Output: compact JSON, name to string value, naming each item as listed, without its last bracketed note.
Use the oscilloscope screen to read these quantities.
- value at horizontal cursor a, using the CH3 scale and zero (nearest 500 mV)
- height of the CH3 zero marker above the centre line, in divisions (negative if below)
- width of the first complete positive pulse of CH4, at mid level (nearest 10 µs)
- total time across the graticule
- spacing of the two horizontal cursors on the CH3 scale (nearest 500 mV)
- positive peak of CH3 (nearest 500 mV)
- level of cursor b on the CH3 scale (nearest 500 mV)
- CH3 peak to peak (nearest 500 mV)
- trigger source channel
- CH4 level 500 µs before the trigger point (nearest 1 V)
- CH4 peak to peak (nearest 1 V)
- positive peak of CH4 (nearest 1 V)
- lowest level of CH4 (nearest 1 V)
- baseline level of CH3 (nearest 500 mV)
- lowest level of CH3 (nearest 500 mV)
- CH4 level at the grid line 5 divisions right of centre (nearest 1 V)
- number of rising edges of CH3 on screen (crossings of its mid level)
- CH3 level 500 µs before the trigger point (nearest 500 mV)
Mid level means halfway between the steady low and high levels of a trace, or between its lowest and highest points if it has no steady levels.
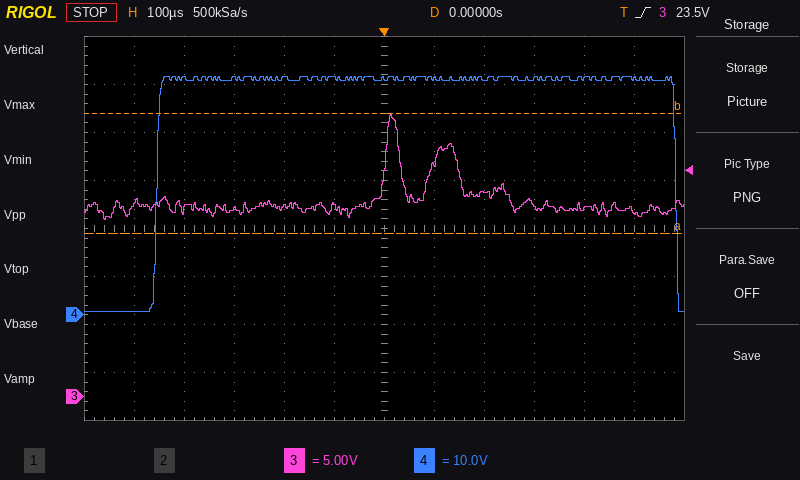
{"value at horizontal cursor a, using the CH3 scale and zero": "17.0 V", "height of the CH3 zero marker above the centre line, in divisions": "-3.5 div", "width of the first complete positive pulse of CH4, at mid level": "1.04 ms", "total time across the graticule": "1.2 ms", "spacing of the two horizontal cursors on the CH3 scale": "12.5 V", "positive peak of CH3": "29.5 V", "level of cursor b on the CH3 scale": "29.5 V", "CH3 peak to peak": "11.0 V", "trigger source channel": "CH3", "CH4 level 500 µs before the trigger point": "1 V", "CH4 peak to peak": "49 V", "positive peak of CH4": "50 V", "lowest level of CH4": "1 V", "baseline level of CH3": "19.5 V", "lowest level of CH3": "18.5 V", "CH4 level at the grid line 5 divisions right of centre": "49 V", "number of rising edges of CH3 on screen": "2", "CH3 level 500 µs before the trigger point": "20.0 V"}
